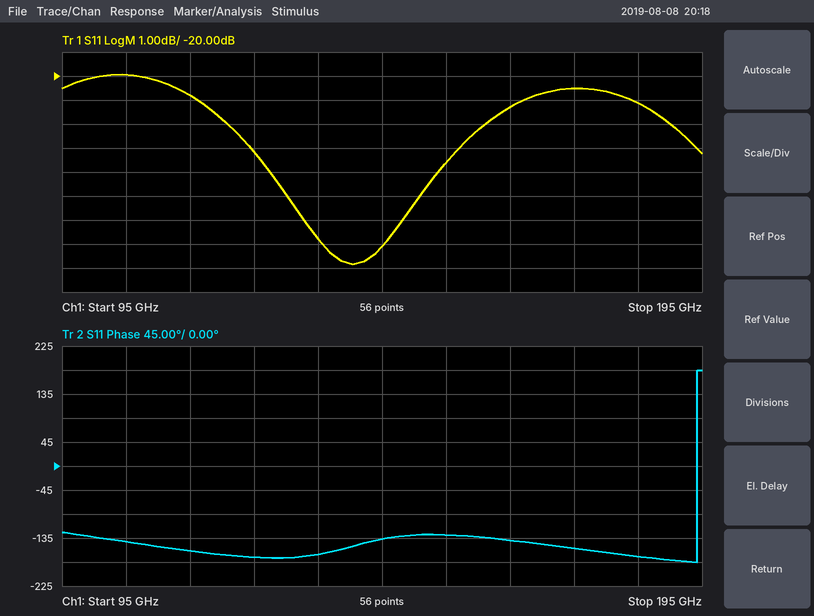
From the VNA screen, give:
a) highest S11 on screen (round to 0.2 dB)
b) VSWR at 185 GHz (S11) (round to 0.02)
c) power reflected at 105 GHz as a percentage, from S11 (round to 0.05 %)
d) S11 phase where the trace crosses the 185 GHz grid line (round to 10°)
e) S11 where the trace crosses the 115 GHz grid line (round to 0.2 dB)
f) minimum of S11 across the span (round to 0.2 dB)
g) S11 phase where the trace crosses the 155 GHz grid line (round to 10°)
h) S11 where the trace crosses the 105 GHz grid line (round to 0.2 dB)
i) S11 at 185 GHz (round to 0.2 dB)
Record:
-20.0 dB
1.20
1.00 %
-170°
-20.8 dB
-27.8 dB
-130°
-20.0 dB
-21.2 dB
